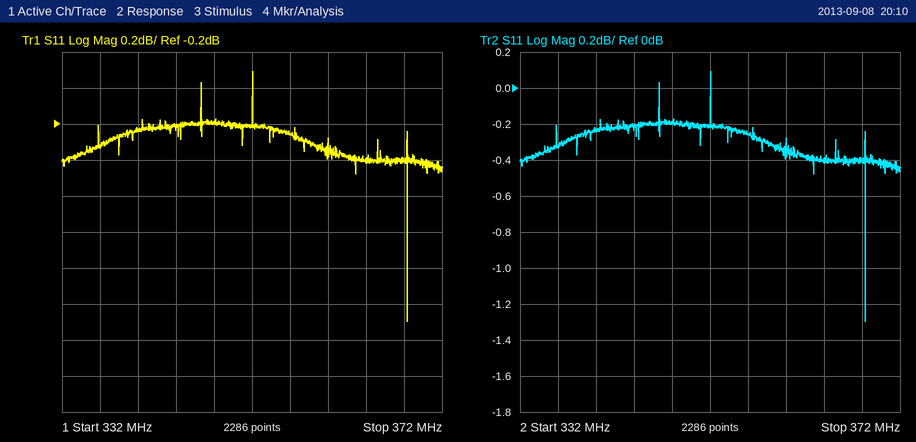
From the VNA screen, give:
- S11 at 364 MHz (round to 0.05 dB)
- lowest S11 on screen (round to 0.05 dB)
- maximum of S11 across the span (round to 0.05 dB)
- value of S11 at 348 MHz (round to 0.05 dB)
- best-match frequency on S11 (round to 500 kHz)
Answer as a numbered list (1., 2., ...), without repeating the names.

1. -0.40 dB
2. -1.30 dB
3. 0.10 dB
4. -0.20 dB
5. 368.5 MHz
